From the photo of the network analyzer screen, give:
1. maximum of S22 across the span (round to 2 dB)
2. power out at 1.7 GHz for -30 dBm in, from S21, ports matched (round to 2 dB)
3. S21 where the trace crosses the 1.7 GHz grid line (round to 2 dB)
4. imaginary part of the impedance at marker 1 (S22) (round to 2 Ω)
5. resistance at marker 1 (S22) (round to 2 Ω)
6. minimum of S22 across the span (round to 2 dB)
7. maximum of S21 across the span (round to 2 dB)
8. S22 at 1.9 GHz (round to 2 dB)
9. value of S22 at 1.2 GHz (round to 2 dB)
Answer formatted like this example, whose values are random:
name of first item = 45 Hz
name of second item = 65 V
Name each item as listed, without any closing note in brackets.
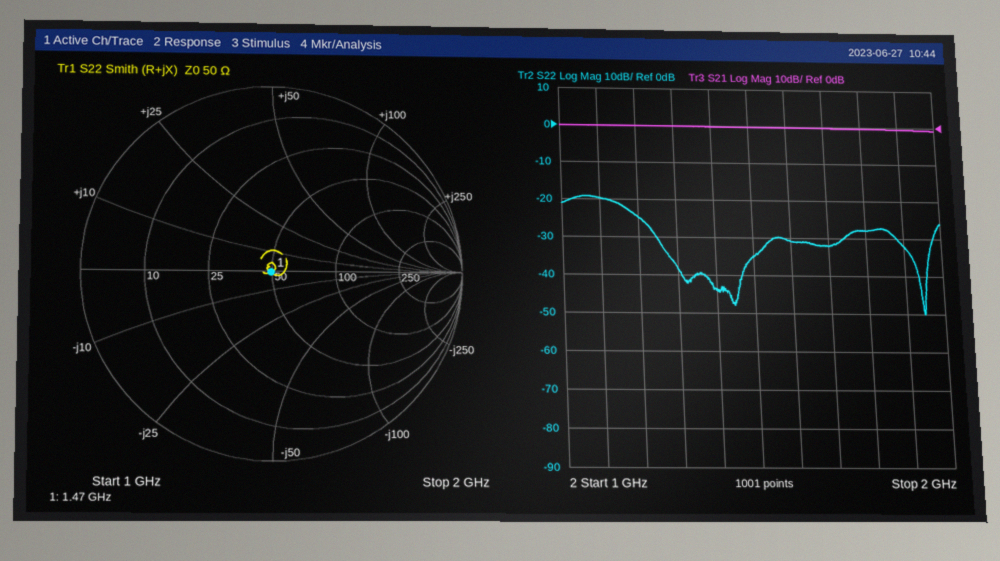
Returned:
maximum of S22 across the span = -20 dB
power out at 1.7 GHz for -30 dBm in, from S21, ports matched = -30 dBm
S21 where the trace crosses the 1.7 GHz grid line = 0 dB
imaginary part of the impedance at marker 1 (S22) = 0 Ω
resistance at marker 1 (S22) = 50 Ω
minimum of S22 across the span = -50 dB
maximum of S21 across the span = 0 dB
S22 at 1.9 GHz = -32 dB
value of S22 at 1.2 GHz = -24 dB
